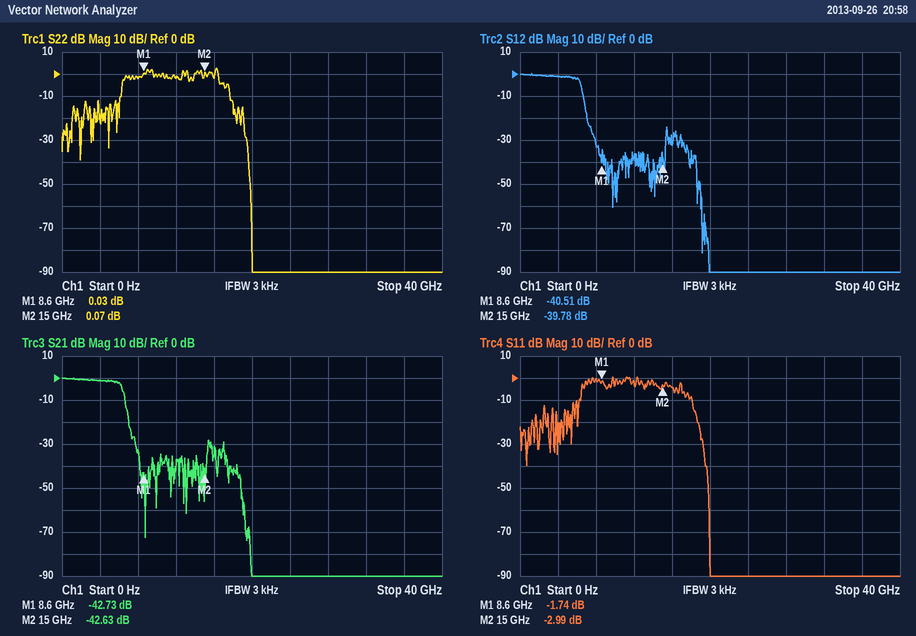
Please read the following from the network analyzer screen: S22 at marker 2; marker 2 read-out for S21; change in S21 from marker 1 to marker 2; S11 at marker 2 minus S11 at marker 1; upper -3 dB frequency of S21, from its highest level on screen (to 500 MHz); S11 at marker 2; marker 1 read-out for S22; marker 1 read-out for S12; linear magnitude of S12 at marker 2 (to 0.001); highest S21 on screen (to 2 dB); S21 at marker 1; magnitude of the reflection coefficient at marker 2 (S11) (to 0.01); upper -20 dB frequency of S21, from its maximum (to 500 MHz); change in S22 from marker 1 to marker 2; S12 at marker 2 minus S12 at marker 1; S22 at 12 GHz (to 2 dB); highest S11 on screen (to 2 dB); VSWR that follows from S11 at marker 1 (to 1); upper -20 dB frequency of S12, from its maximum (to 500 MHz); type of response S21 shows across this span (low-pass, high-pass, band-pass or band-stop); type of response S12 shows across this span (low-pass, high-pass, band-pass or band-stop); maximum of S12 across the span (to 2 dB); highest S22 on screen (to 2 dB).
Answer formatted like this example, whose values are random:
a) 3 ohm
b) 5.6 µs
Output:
a) 0.07 dB
b) -42.63 dB
c) 0.10 dB
d) -1.25 dB
e) 6.0 GHz
f) -2.99 dB
g) 0.03 dB
h) -40.51 dB
i) 0.010
j) 0 dB
k) -42.73 dB
l) 0.71
m) 7.0 GHz
n) 0.04 dB
o) 0.73 dB
p) -2 dB
q) 0 dB
r) 10
s) 7.0 GHz
t) low-pass
u) low-pass
v) 0 dB
w) 2 dB
